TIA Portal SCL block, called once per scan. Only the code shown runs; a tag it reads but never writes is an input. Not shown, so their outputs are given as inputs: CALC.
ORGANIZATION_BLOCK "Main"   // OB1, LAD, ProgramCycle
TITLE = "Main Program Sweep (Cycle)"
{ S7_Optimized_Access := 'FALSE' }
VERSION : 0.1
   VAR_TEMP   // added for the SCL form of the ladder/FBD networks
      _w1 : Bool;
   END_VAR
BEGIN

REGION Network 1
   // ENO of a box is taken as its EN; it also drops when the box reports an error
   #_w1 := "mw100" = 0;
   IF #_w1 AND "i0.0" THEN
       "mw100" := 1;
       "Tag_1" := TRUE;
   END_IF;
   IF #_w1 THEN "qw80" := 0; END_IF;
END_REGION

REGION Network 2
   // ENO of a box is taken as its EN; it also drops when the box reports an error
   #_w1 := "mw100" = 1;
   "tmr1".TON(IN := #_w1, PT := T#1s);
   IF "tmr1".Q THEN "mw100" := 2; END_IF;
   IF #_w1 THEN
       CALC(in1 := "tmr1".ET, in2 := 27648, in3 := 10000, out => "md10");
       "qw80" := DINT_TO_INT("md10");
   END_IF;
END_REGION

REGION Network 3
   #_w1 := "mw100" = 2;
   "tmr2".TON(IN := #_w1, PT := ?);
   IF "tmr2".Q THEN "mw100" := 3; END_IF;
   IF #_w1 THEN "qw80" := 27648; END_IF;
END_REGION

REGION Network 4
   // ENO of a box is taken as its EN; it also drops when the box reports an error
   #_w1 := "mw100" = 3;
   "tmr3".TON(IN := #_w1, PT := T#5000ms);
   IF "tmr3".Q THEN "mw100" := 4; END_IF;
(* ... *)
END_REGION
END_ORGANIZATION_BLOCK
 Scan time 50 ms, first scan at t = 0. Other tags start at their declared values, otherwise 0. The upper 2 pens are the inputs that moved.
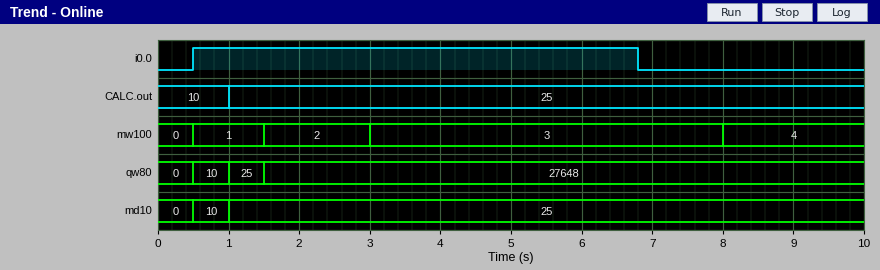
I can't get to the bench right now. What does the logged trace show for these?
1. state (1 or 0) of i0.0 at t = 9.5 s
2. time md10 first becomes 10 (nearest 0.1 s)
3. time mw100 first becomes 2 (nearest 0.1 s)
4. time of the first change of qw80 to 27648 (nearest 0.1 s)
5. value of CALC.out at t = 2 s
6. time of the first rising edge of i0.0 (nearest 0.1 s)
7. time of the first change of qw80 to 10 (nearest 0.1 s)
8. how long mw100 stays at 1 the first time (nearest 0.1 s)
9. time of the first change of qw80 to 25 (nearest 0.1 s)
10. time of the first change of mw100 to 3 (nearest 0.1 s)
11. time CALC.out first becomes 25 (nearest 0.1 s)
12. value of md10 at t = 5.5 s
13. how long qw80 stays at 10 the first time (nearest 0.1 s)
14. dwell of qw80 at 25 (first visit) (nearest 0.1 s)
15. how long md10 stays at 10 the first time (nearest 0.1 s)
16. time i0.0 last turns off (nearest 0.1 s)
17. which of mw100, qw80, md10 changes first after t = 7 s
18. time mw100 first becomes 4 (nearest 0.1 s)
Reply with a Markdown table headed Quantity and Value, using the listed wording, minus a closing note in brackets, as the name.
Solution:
| Quantity | Value |
|---|---|
| state (1 or 0) of i0.0 at t = 9.5 s | 0 |
| time md10 first becomes 10 | 0.5 s |
| time mw100 first becomes 2 | 1.5 s |
| time of the first change of qw80 to 27648 | 1.5 s |
| value of CALC.out at t = 2 s | 25 |
| time of the first rising edge of i0.0 | 0.5 s |
| time of the first change of qw80 to 10 | 0.5 s |
| how long mw100 stays at 1 the first time | 1.0 s |
| time of the first change of qw80 to 25 | 1.0 s |
| time of the first change of mw100 to 3 | 3.0 s |
| time CALC.out first becomes 25 | 1.0 s |
| value of md10 at t = 5.5 s | 25 |
| how long qw80 stays at 10 the first time | 0.5 s |
| dwell of qw80 at 25 (first visit) | 0.5 s |
| how long md10 stays at 10 the first time | 0.5 s |
| time i0.0 last turns off | 6.8 s |
| which of mw100, qw80, md10 changes first after t = 7 s | mw100 |
| time mw100 first becomes 4 | 8.0 s |
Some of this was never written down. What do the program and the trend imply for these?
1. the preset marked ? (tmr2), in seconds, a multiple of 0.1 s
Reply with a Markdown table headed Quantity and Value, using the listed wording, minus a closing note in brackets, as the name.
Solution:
| Quantity | Value |
|---|---|
| the preset marked ? (tmr2), in seconds, a multiple of 0.1 s | 1.5 s |
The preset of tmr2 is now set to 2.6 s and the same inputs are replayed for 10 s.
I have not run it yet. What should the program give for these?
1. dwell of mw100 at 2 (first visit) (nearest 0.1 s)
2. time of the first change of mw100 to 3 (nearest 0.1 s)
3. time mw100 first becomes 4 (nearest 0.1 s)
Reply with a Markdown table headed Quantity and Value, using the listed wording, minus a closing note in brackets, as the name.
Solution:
| Quantity | Value |
|---|---|
| dwell of mw100 at 2 (first visit) | 2.6 s |
| time of the first change of mw100 to 3 | 4.1 s |
| time mw100 first becomes 4 | 9.1 s |
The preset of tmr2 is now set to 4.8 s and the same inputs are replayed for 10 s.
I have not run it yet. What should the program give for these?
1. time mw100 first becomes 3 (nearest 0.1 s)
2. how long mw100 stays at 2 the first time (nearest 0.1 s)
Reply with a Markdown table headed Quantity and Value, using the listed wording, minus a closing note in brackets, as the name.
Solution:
| Quantity | Value |
|---|---|
| time mw100 first becomes 3 | 6.3 s |
| how long mw100 stays at 2 the first time | 4.8 s |
